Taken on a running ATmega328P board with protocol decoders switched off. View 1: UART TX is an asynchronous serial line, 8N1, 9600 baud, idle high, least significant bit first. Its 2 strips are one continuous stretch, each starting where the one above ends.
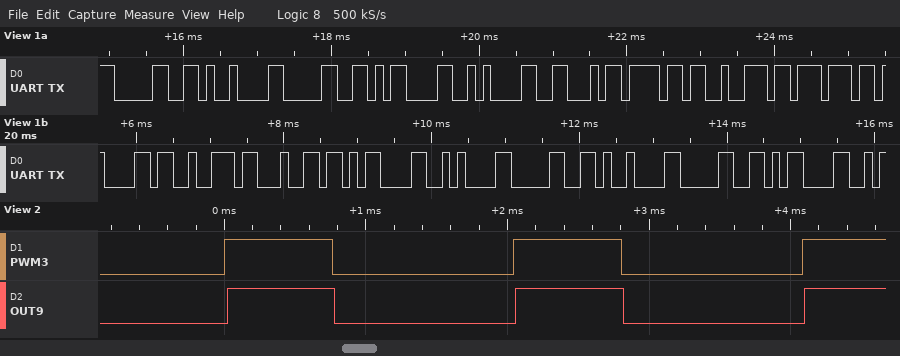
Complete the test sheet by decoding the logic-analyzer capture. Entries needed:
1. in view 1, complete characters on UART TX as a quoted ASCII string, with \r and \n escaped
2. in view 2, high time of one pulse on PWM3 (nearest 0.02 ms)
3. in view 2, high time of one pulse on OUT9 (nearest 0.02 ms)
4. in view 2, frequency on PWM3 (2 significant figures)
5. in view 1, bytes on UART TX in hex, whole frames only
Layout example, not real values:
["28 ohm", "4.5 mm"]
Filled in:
["\"0\\t0\\r\\nForward\\r\\n0\\t0\\r\"", "0.76 ms", "0.76 ms", "490 Hz", "30 09 30 0D 0A 46 6F 72 77 61 72 64 0D 0A 30 09 30 0D"]
